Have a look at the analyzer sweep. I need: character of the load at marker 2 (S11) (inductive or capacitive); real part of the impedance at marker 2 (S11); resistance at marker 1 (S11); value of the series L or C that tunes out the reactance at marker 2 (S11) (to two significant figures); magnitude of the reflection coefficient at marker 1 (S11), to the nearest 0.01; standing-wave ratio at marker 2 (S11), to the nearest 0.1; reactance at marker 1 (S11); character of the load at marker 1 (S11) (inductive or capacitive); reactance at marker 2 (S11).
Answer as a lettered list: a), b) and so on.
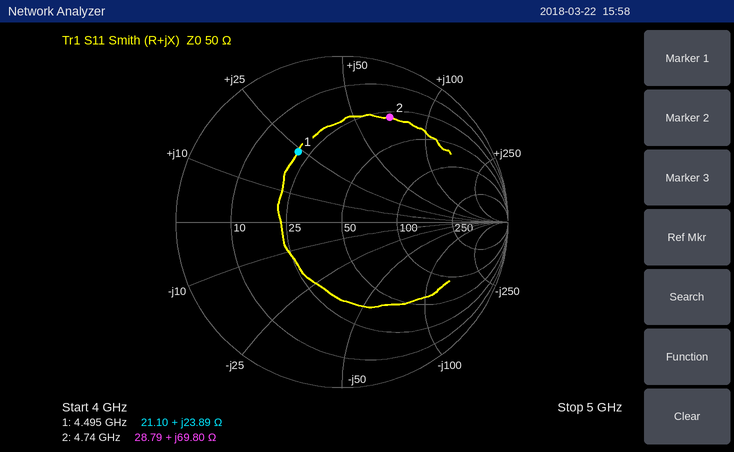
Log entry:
a) inductive
b) 28.79 Ω
c) 21.10 Ω
d) 480 fF
e) 0.50
f) 5.5
g) +23.89 Ω
h) inductive
i) +69.80 Ω
